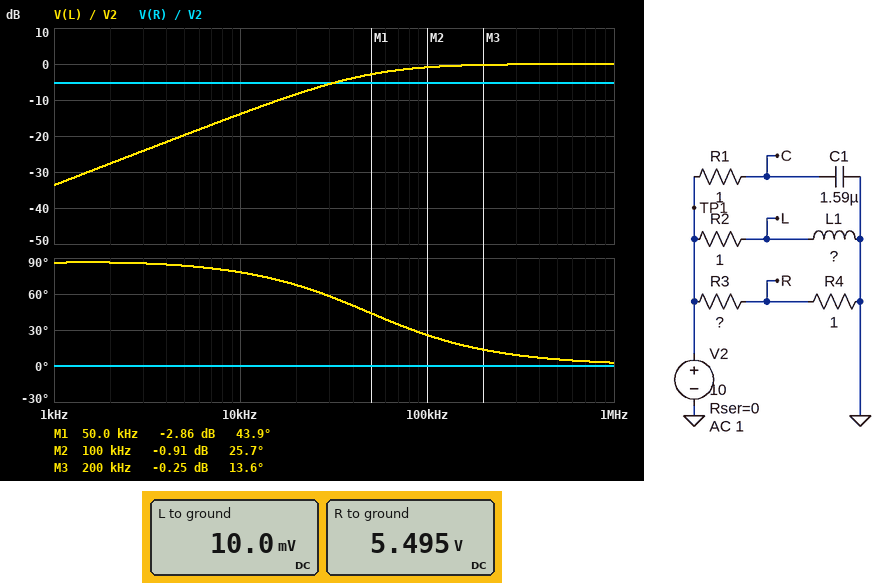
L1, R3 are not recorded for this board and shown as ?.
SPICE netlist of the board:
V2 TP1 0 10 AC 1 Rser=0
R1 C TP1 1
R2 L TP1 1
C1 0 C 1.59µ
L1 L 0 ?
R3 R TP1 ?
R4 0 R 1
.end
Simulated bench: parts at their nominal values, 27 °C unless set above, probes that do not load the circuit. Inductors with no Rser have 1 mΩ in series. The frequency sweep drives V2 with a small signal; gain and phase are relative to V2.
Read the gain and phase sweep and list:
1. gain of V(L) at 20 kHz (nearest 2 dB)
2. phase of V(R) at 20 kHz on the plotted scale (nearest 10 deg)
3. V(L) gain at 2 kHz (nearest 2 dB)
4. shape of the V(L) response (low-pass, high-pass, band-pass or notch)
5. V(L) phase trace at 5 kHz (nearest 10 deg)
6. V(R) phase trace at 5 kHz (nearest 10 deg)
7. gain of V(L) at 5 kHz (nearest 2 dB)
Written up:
-8 dB
0 deg
-28 dB
high-pass
80 deg
0 deg
-20 dB
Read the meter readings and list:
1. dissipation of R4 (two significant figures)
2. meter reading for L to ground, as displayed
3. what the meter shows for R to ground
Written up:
30 W
10.0 mV
5.495 V
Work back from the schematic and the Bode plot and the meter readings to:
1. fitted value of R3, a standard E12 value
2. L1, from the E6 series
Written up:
0.82 Ω
3.3 µH
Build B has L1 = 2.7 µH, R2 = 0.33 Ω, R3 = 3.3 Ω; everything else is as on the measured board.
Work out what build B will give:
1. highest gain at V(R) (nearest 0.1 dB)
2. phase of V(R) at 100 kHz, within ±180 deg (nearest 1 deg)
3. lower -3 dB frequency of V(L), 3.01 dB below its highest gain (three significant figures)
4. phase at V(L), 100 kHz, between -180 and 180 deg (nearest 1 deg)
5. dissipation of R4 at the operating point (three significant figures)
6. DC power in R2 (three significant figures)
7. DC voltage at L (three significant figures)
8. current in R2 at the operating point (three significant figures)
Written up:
-12.7 dB
0 deg
19.5 kHz
11 deg
5.41 W
301 W
30.2 mV
30.2 A
